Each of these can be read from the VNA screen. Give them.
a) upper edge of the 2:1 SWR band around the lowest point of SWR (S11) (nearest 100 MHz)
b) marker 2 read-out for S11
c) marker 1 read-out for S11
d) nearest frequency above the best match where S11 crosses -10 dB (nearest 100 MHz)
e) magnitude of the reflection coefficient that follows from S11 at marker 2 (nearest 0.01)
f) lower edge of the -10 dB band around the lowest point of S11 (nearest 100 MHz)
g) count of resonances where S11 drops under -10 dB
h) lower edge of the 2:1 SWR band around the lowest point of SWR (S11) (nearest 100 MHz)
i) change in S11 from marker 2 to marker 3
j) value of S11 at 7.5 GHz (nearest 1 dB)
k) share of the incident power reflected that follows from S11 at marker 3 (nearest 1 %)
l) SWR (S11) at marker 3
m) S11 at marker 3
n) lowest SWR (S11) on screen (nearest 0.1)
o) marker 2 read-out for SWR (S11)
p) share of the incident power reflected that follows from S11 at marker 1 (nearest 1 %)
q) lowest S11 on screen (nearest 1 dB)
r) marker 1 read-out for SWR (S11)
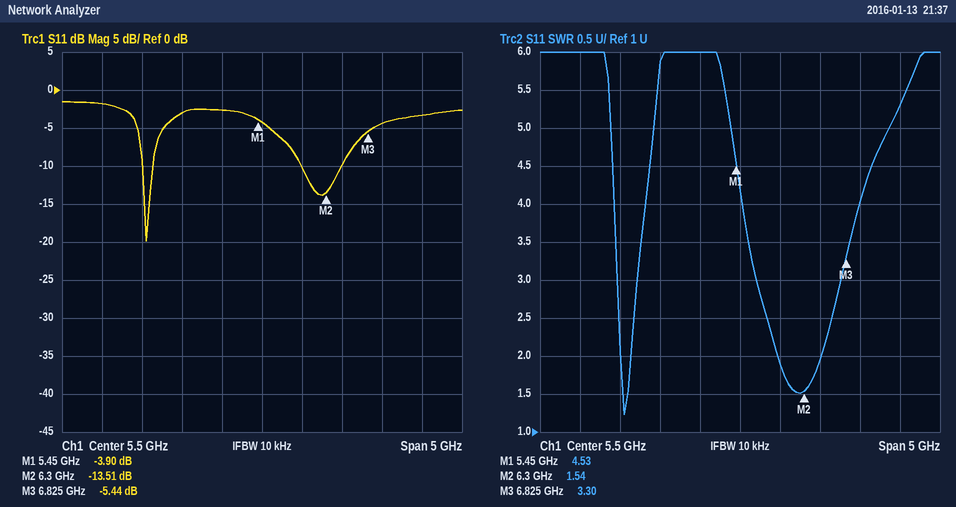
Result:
4.1 GHz
-13.51 dB
-3.90 dB
4.1 GHz
0.21
4.0 GHz
2
4.0 GHz
8.07 dB
-3 dB
29 %
3.30
-5.44 dB
1.2
1.54
41 %
-20 dB
4.53
